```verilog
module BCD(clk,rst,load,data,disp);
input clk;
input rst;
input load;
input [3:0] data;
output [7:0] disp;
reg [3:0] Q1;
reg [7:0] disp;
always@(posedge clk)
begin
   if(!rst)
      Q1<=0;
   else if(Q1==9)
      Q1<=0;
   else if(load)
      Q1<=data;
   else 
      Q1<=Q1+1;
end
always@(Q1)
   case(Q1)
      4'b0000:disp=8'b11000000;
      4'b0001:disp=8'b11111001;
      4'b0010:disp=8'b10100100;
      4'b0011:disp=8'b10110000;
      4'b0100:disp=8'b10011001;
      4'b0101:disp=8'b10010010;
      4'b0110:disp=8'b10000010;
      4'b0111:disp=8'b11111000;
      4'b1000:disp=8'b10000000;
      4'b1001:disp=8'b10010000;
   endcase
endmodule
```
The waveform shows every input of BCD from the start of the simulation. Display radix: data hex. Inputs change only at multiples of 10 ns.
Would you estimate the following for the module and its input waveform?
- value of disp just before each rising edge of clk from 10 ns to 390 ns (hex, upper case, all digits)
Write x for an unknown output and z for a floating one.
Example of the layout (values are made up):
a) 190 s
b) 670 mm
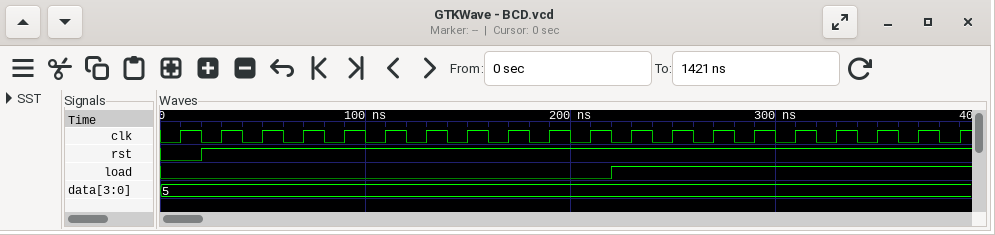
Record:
a) x, C0, F9, A4, B0, 99, 92, 82, F8, 80, 90, C0, 92, 92, 92, 92, 92, 92, 92, 92
